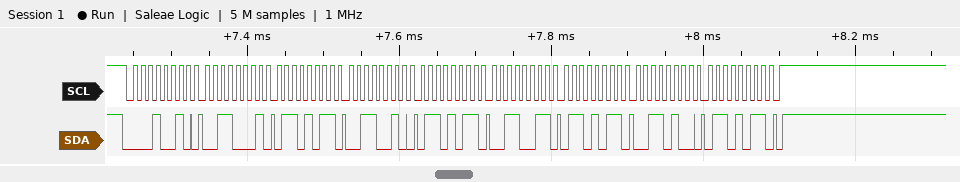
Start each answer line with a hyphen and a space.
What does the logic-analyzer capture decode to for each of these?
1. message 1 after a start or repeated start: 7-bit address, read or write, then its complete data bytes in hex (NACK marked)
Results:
- 0x09 write: 31 6B 32 6B 33 6B 34 6B
